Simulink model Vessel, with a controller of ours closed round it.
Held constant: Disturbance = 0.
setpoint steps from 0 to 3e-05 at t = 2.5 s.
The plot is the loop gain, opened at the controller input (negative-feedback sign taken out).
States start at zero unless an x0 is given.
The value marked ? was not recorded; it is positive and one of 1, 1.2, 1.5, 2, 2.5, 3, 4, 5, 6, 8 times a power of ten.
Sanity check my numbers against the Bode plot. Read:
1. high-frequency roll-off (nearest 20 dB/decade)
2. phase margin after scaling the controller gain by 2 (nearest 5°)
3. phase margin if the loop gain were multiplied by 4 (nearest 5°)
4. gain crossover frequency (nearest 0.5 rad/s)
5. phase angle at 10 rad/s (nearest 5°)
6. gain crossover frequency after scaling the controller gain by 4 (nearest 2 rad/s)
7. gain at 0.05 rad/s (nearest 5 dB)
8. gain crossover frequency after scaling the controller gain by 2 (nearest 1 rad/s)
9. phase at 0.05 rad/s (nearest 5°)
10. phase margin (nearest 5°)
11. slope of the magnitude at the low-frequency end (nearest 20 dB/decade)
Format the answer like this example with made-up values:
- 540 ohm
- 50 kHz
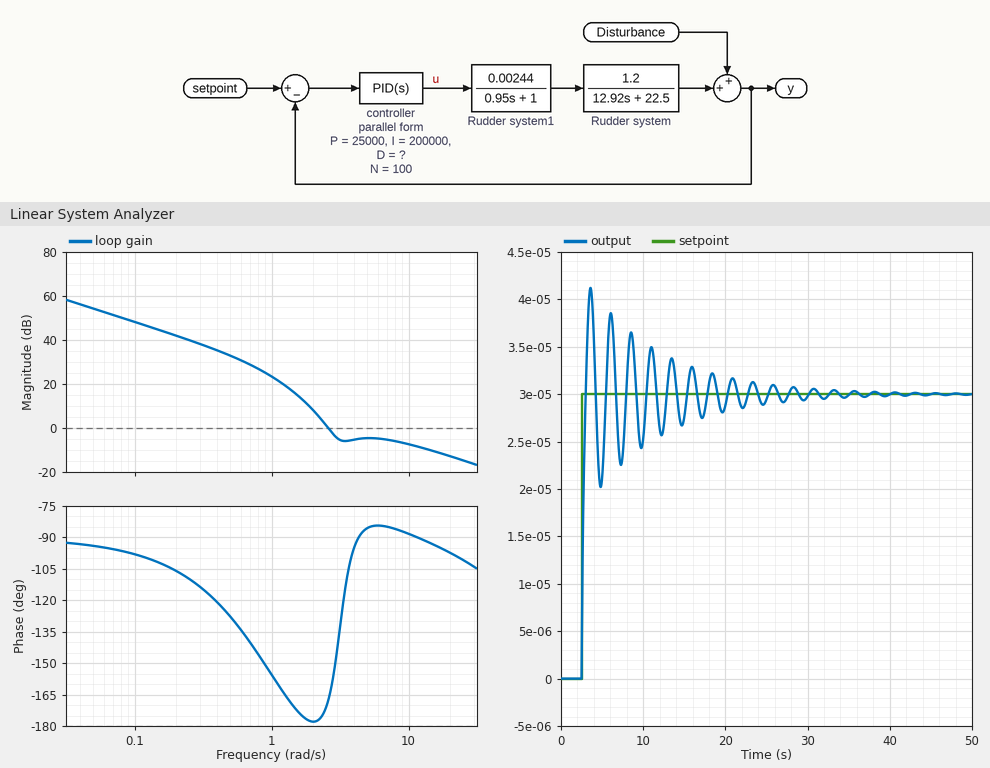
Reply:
- -20 dB/decade
- 95°
- 85°
- 2.5 rad/s
- -90°
- 18 rad/s
- 55 dB
- 8 rad/s
- -95°
- 10°
- -20 dB/decade
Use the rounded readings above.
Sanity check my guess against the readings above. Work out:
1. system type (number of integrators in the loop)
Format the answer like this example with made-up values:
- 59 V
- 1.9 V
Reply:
- 1
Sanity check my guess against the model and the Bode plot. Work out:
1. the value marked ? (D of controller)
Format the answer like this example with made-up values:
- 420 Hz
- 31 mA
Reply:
- 20000
